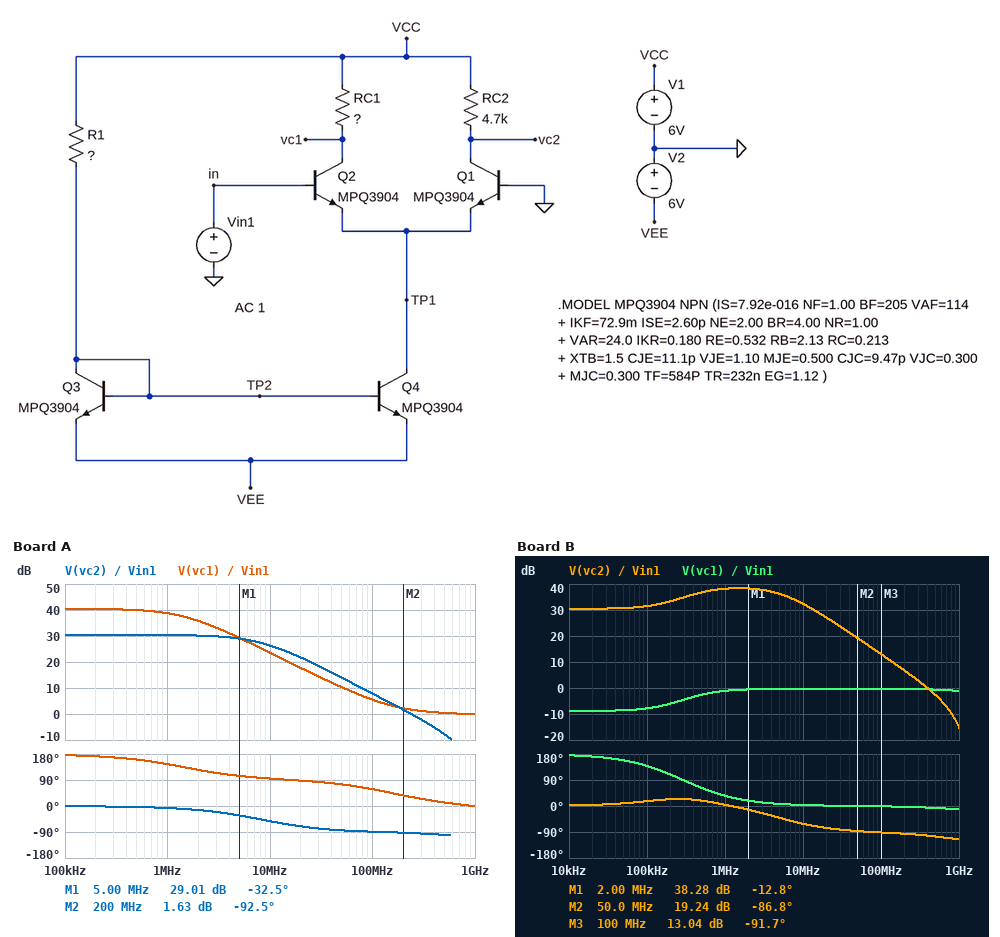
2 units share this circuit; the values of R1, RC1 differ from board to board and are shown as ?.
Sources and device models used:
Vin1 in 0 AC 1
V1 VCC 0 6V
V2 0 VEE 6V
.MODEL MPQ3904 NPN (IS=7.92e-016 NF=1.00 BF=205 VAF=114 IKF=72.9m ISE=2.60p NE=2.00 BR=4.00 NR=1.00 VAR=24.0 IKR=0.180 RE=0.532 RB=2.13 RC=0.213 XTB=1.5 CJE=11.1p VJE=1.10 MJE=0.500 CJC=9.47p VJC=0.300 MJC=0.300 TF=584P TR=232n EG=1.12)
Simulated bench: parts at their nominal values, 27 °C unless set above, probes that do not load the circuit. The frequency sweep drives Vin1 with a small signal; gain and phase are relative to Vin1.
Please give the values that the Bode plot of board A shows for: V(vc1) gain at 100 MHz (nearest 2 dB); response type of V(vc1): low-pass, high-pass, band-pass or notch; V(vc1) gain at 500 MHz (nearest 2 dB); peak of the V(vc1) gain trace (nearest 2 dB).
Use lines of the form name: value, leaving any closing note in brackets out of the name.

V(vc1) gain at 100 MHz: 6 dB
response type of V(vc1): low-pass, high-pass, band-pass or notch: low-pass
V(vc1) gain at 500 MHz: 0 dB
peak of the V(vc1) gain trace: 40 dB
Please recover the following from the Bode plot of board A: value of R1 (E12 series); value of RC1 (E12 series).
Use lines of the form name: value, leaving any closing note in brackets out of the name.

value of R1: 15 kΩ
value of RC1: 15 kΩ
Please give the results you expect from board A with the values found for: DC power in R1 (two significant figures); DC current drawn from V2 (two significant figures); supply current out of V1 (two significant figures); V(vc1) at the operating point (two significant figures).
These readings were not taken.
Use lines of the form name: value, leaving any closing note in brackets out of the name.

DC power in R1: 8.5 mW
DC current drawn from V2: 1.5 mA
supply current out of V1: 1.5 mA
V(vc1) at the operating point: 380 mV
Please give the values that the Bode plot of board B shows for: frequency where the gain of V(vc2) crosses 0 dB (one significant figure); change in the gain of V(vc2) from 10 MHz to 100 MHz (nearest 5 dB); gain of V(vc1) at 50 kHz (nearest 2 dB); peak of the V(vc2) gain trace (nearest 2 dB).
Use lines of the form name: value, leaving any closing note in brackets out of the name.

frequency where the gain of V(vc2) crosses 0 dB: 400 MHz
change in the gain of V(vc2) from 10 MHz to 100 MHz: -20 dB
gain of V(vc1) at 50 kHz: -8 dB
peak of the V(vc2) gain trace: 38 dB
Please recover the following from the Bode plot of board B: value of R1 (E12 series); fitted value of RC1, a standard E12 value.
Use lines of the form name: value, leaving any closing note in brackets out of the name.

value of R1: 6.8 kΩ
fitted value of RC1, a standard E12 value: 15 kΩ
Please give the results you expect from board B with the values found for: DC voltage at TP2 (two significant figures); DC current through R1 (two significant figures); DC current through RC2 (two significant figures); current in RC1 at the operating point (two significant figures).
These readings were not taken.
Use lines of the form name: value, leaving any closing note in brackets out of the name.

DC voltage at TP2: -5.3 V
DC current through R1: 1.7 mA
DC current through RC2: 1.1 mA
current in RC1 at the operating point: 450 µA
